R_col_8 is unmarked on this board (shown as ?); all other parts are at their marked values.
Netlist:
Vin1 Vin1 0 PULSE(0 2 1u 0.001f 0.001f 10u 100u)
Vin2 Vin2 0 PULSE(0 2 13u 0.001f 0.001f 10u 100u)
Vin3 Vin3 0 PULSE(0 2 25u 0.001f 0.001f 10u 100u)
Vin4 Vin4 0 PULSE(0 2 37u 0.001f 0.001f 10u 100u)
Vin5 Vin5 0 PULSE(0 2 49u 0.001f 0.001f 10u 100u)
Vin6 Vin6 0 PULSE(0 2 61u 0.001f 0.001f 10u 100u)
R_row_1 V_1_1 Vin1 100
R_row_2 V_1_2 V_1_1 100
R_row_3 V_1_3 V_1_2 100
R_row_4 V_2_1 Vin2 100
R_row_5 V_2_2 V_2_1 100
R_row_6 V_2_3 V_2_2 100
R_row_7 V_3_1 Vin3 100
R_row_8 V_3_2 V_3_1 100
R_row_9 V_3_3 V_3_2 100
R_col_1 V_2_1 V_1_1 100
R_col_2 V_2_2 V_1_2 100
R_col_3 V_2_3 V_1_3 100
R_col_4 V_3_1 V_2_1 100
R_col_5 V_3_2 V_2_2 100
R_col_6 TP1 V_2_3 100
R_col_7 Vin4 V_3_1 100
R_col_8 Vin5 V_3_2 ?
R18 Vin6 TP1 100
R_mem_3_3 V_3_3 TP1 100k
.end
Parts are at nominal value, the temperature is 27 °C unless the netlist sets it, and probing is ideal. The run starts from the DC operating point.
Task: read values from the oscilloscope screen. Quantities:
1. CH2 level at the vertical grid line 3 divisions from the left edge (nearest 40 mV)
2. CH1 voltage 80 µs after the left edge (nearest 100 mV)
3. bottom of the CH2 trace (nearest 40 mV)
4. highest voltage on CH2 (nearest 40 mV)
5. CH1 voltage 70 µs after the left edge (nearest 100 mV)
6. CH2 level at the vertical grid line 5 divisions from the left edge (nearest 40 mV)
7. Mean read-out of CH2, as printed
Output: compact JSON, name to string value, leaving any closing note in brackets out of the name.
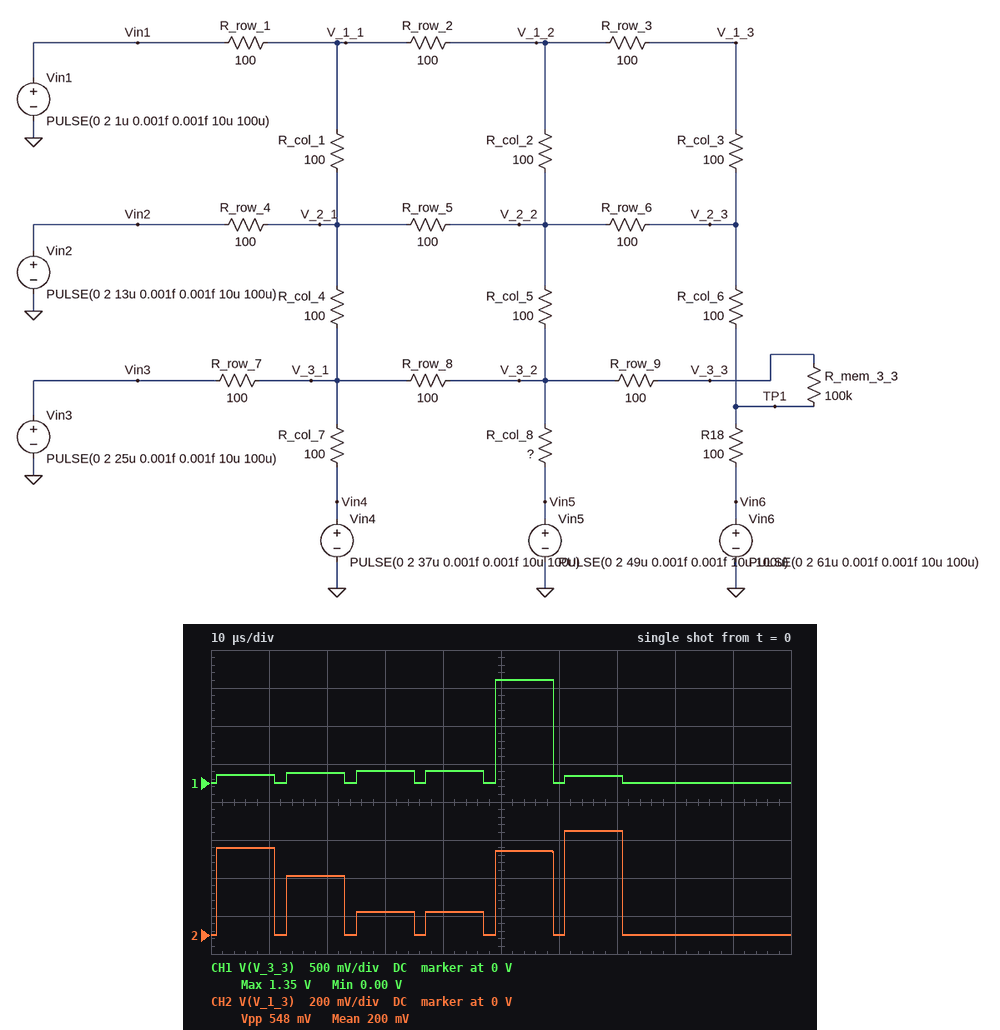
{"CH2 level at the vertical grid line 3 divisions from the left edge": "120 mV", "CH1 voltage 80 µs after the left edge": "0 V", "bottom of the CH2 trace": "0 V", "highest voltage on CH2": "560 mV", "CH1 voltage 70 µs after the left edge": "100 mV", "CH2 level at the vertical grid line 5 divisions from the left edge": "440 mV", "Mean read-out of CH2, as printed": "200 mV"}
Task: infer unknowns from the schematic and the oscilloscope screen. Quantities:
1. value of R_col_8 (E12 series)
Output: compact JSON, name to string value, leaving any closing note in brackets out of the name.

{"value of R_col_8": "39 Ω"}
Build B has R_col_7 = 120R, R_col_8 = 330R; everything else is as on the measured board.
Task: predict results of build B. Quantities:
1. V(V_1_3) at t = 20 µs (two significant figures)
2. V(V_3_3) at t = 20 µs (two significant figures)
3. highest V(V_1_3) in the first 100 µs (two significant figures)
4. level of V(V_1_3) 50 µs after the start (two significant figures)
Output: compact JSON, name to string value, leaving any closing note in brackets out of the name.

{"V(V_1_3) at t = 20 µs": "380 mV", "V(V_3_3) at t = 20 µs": "330 mV", "highest V(V_1_3) in the first 100 µs": "590 mV", "level of V(V_1_3) 50 µs after the start": "130 mV"}
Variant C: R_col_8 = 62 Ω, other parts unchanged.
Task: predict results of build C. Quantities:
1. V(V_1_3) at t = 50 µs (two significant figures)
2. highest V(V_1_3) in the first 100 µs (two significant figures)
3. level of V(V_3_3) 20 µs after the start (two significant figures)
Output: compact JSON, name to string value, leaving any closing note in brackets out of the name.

{"V(V_1_3) at t = 50 µs": "370 mV", "highest V(V_1_3) in the first 100 µs": "560 mV", "level of V(V_3_3) 20 µs after the start": "170 mV"}
